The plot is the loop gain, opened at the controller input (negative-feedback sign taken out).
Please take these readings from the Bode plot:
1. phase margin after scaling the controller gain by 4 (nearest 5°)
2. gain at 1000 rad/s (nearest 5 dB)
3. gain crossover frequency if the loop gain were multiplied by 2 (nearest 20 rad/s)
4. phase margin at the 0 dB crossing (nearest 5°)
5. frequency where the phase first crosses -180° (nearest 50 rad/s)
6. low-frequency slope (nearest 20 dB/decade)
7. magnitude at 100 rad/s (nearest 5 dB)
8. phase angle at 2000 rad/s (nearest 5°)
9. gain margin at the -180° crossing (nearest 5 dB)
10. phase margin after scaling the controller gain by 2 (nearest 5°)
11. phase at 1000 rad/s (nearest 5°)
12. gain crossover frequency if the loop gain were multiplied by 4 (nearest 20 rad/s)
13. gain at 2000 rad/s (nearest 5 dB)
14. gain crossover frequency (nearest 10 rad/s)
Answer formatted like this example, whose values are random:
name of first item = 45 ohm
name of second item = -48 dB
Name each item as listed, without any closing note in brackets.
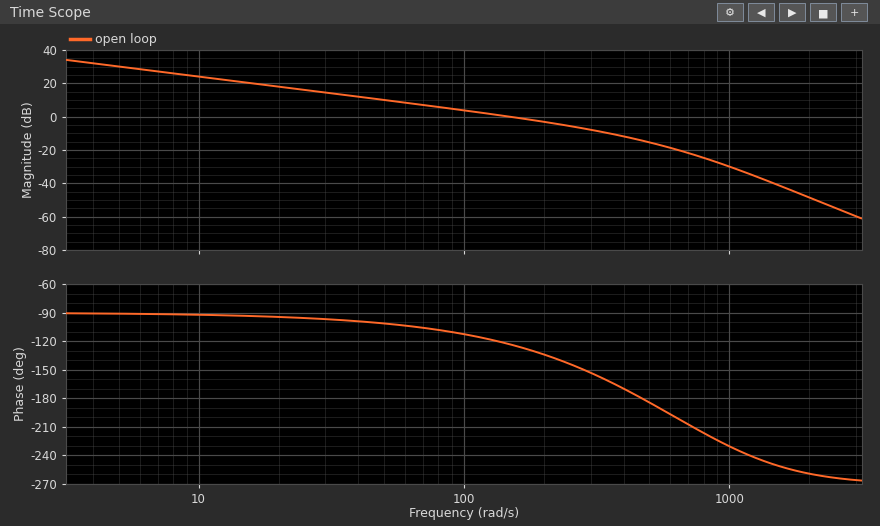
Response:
phase margin after scaling the controller gain by 4 = 10°
gain at 1000 rad/s = -30 dB
gain crossover frequency if the loop gain were multiplied by 2 = 260 rad/s
phase margin at the 0 dB crossing = 55°
frequency where the phase first crosses -180° = 450 rad/s
low-frequency slope = -20 dB/decade
magnitude at 100 rad/s = 5 dB
phase angle at 2000 rad/s = -260°
gain margin at the -180° crossing = 15 dB
phase margin after scaling the controller gain by 2 = 35°
phase at 1000 rad/s = -230°
gain crossover frequency if the loop gain were multiplied by 4 = 400 rad/s
gain at 2000 rad/s = -50 dB
gain crossover frequency = 150 rad/s
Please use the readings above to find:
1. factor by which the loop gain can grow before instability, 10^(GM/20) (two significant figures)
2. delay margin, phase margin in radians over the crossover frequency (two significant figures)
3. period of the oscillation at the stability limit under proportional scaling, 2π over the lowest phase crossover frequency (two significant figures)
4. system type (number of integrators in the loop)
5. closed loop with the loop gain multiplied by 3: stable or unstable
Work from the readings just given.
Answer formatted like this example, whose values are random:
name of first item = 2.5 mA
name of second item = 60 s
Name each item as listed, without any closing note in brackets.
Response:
factor by which the loop gain can grow before instability, 10^(GM/20) = 5.6
delay margin, phase margin in radians over the crossover frequency = 0.0064 s
period of the oscillation at the stability limit under proportional scaling, 2π over the lowest phase crossover frequency = 0.014 s
system type = 1
closed loop with the loop gain multiplied by 3: stable or unstable = stable
